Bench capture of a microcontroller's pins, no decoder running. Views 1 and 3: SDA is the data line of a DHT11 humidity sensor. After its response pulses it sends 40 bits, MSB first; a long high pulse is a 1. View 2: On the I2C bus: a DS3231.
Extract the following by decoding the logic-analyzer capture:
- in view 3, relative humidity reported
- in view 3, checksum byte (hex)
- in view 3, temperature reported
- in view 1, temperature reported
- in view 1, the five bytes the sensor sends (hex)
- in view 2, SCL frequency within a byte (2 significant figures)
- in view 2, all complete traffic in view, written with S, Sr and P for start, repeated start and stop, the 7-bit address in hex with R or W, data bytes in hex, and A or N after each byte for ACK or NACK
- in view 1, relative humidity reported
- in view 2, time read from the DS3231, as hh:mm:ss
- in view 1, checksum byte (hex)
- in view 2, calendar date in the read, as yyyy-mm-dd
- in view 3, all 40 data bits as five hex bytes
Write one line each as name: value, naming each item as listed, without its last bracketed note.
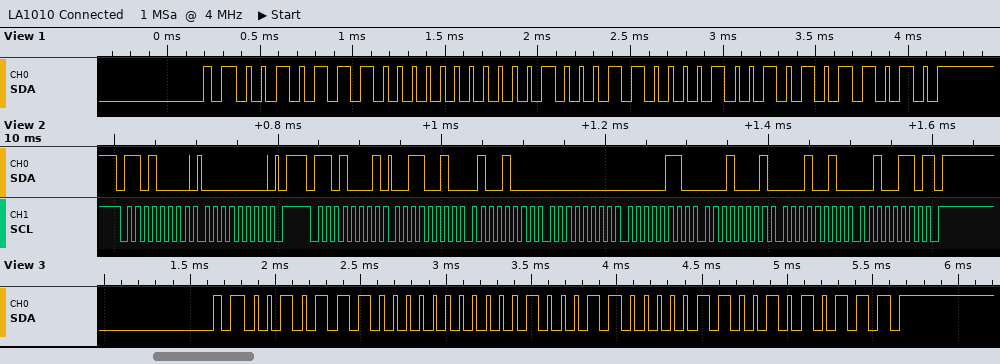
in view 3, relative humidity reported: 46 %
in view 3, checksum byte: 0x57
in view 3, temperature reported: 35.6 °C
in view 1, temperature reported: 35.9 °C
in view 1, the five bytes the sensor sends: 2E 00 23 09 5A
in view 2, SCL frequency within a byte: 100 kHz
in view 2, all complete traffic in view, written with S, Sr and P for start, repeated start and stop, the 7-bit address in hex with R or W, data bytes in hex, and A or N after each byte for ACK or NACK: S 68W A 00 A P S 68R A 32 A 48 A 00 A 06 A 11 A 12 A 26 N P
in view 1, relative humidity reported: 46 %
in view 2, time read from the DS3231, as hh:mm:ss: 00:48:32
in view 1, checksum byte: 0x5A
in view 2, calendar date in the read, as yyyy-mm-dd: 2026-12-11
in view 3, all 40 data bits as five hex bytes: 2E 00 23 06 57
